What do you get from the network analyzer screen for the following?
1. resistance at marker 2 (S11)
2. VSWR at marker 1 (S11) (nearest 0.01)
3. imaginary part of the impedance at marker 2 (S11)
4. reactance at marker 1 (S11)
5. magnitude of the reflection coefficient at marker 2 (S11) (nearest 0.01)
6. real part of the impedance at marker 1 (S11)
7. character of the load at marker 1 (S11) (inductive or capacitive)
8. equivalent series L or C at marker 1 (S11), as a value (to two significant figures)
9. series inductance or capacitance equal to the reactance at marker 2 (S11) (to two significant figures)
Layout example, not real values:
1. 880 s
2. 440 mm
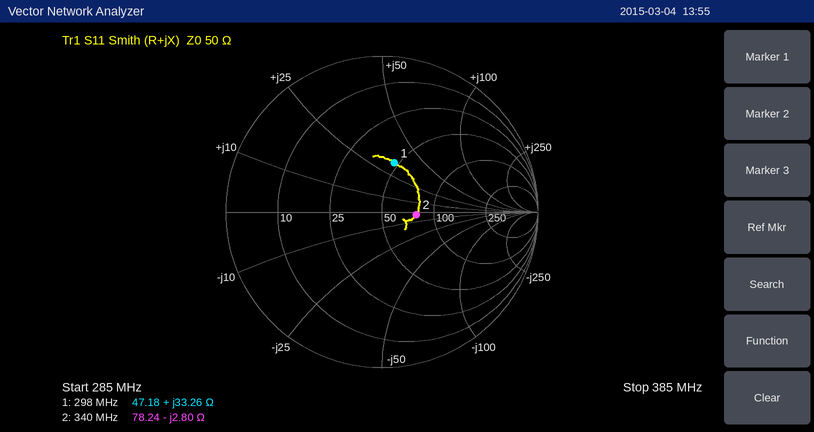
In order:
1. 78.24 Ω
2. 1.96
3. -2.80 Ω
4. +33.26 Ω
5. 0.22
6. 47.18 Ω
7. inductive
8. 18 nH
9. 170 pF
